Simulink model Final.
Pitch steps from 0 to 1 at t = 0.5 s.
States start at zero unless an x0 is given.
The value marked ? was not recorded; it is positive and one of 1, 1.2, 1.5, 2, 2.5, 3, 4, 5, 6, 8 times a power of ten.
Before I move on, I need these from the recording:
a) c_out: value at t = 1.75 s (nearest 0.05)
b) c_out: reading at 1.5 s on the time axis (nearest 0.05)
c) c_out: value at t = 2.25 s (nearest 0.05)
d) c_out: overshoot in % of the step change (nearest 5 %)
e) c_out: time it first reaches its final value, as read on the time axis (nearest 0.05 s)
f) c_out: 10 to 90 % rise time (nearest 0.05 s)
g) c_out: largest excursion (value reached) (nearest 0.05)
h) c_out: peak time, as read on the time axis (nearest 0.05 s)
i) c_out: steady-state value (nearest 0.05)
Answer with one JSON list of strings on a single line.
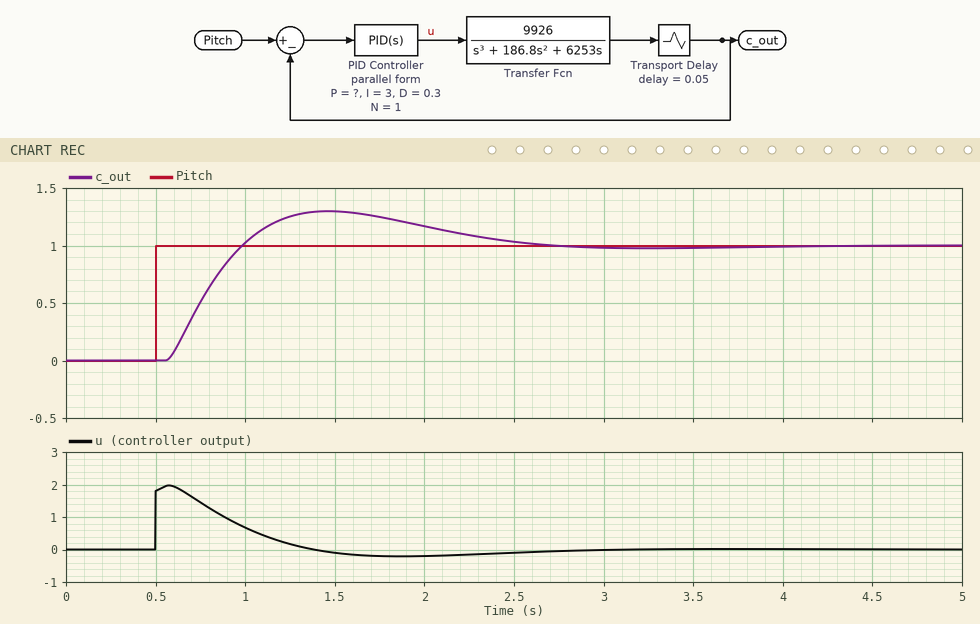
["1.25", "1.30", "1.10", "30 %", "1.00 s", "0.30 s", "1.30", "1.45 s", "1.00"]
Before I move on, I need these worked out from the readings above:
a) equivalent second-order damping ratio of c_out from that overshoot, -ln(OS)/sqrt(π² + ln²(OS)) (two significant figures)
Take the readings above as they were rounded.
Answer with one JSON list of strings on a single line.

["0.36"]
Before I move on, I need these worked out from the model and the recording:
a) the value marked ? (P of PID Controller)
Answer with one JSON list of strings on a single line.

["1.5"]
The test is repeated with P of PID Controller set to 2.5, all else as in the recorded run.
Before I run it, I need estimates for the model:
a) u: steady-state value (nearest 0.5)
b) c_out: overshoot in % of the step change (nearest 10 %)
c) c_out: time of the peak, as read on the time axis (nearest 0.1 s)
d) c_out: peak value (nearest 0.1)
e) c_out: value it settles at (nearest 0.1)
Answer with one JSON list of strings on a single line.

["0.0", "20 %", "1.2 s", "1.2", "1.0"]
